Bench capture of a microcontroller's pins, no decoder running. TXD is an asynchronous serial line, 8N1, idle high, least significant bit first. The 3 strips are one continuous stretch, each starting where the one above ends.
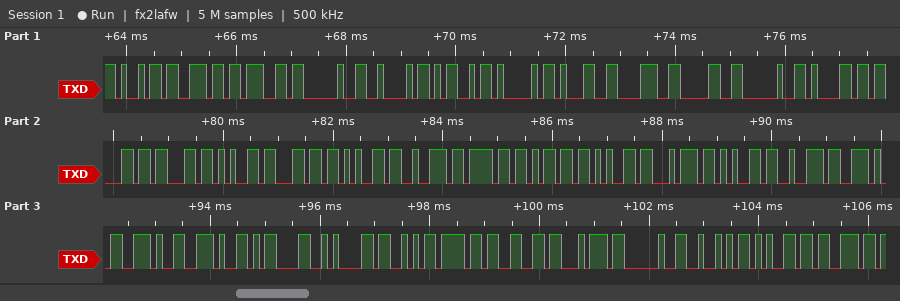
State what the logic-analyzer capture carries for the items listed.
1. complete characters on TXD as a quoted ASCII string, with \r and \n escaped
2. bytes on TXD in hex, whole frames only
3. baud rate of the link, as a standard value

"ing BMA180 accelerometer...\r\nSoft Res"
69 6E 67 20 42 4D 41 31 38 30 20 61 63 63 65 6C 65 72 6F 6D 65 74 65 72 2E 2E 2E 0D 0A 53 6F 66 74 20 52 65 73
9600 baud
